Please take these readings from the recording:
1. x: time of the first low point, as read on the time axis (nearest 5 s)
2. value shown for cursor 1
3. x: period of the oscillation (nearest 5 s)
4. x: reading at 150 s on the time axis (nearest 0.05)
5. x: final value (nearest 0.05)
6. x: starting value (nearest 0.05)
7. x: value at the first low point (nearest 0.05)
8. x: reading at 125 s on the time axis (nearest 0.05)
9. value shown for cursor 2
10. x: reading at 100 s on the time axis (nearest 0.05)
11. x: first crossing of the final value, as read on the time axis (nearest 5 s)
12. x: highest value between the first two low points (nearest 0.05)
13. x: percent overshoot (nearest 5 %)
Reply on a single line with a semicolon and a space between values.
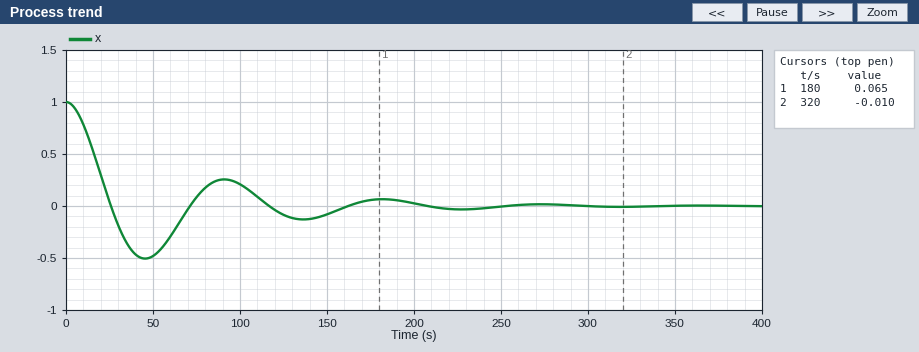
45 s; 0.065; 90 s; -0.10; 0.00; 1.00; -0.50; -0.10; -0.010; 0.20; 25 s; 0.25; 50 %
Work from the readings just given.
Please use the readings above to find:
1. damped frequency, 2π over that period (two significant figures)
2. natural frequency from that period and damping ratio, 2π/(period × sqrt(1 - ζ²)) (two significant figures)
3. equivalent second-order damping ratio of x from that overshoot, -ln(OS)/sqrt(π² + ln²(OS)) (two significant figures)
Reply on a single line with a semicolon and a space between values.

0.070 rad/s; 0.072 rad/s; 0.22
